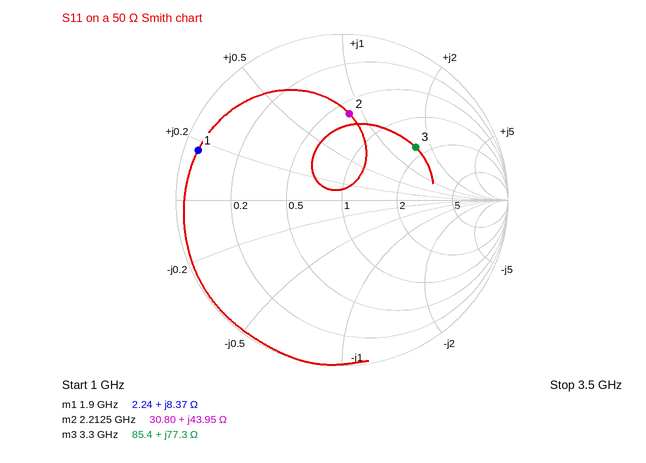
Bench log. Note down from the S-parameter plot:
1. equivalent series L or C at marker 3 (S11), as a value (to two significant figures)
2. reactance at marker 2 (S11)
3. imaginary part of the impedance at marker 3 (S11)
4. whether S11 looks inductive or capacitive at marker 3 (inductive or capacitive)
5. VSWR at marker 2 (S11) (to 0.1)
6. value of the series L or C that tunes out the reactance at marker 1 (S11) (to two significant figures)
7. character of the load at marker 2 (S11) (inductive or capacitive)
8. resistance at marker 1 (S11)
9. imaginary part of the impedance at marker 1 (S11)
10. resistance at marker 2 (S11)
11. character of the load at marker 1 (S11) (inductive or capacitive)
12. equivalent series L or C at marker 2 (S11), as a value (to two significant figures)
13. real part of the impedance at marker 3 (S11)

3.7 nH
+43.95 Ω
+77.3 Ω
inductive
3.2
10 pF
inductive
2.24 Ω
+8.37 Ω
30.80 Ω
inductive
3.2 nH
85.4 Ω
